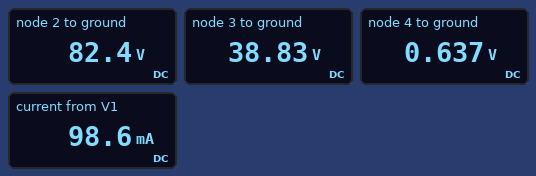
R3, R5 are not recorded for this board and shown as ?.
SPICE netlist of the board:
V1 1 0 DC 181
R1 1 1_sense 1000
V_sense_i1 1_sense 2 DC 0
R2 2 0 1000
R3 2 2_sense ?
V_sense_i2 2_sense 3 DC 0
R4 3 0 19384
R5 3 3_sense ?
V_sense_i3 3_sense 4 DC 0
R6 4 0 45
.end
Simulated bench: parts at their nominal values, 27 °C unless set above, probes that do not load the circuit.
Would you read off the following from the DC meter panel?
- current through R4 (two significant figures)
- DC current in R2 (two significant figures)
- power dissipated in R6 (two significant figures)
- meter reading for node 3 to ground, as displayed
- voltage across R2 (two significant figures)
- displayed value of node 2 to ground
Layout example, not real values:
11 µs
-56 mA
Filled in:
2.0 mA
82 mA
9.0 mW
38.83 V
82 V
82.4 V
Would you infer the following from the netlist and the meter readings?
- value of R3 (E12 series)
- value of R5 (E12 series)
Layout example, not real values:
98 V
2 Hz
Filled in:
2.7 kΩ
2.7 kΩ
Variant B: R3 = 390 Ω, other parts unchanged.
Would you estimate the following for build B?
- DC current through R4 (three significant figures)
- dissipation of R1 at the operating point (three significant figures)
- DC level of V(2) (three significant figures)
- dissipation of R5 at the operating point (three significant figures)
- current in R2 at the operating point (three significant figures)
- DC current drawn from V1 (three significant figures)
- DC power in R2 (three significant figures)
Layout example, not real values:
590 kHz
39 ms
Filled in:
3.41 mA
10.9 W
76.8 V
1.56 W
76.8 mA
104 mA
5.89 W
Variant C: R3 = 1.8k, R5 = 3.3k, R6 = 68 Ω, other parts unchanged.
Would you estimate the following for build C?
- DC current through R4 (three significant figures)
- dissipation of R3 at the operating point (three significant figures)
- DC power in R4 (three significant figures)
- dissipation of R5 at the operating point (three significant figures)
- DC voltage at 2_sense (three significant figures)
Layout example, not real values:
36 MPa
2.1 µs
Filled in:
2.59 mA
552 mW
130 mW
734 mW
50.2 V
